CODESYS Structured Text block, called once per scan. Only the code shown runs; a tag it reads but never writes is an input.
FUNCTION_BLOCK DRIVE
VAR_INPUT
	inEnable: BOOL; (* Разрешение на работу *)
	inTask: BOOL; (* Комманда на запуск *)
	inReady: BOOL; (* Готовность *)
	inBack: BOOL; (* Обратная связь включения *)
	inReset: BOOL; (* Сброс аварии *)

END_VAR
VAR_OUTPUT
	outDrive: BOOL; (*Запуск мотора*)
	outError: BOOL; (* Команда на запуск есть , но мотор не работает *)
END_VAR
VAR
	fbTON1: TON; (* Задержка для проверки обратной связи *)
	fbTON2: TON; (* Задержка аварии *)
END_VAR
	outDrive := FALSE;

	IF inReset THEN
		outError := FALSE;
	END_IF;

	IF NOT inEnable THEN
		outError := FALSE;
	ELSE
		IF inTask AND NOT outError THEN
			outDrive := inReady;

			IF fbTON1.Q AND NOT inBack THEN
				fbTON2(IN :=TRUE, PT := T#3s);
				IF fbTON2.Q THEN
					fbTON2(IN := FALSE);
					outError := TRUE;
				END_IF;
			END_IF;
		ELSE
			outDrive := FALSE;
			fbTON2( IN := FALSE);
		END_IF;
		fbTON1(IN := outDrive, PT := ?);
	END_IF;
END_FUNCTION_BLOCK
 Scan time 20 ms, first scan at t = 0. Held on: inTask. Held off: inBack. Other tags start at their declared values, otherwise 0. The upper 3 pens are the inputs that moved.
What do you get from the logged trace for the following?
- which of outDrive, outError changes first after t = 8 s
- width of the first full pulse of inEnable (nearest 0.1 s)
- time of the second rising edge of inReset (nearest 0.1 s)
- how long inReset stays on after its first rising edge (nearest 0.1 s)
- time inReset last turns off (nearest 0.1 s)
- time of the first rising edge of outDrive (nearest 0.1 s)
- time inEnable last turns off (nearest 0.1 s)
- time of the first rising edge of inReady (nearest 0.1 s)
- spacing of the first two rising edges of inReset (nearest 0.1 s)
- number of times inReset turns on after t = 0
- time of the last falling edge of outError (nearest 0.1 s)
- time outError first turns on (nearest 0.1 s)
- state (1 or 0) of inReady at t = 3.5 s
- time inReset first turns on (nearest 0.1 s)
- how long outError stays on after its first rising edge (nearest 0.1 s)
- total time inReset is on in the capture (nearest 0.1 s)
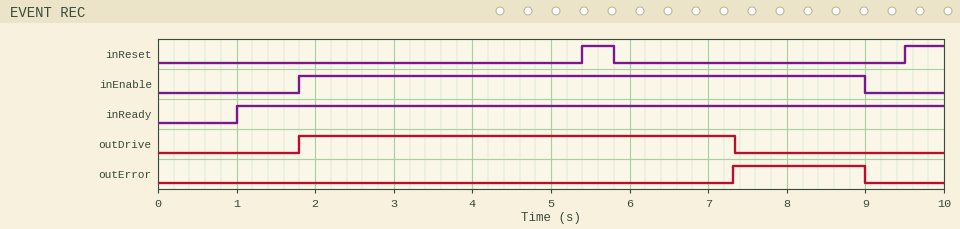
outError
7.2 s
9.5 s
0.4 s
5.8 s
1.8 s
9.0 s
1.0 s
4.1 s
2
9.0 s
7.3 s
1
5.4 s
1.7 s
0.9 s
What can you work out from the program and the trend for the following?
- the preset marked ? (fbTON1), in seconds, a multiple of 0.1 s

2.5 s
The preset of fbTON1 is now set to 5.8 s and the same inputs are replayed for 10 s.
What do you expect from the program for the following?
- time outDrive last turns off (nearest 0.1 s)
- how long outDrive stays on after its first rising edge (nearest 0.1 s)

9.0 s
7.2 s
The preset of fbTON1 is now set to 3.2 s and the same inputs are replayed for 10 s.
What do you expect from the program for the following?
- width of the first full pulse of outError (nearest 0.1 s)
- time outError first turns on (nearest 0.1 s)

1.0 s
8.0 s
